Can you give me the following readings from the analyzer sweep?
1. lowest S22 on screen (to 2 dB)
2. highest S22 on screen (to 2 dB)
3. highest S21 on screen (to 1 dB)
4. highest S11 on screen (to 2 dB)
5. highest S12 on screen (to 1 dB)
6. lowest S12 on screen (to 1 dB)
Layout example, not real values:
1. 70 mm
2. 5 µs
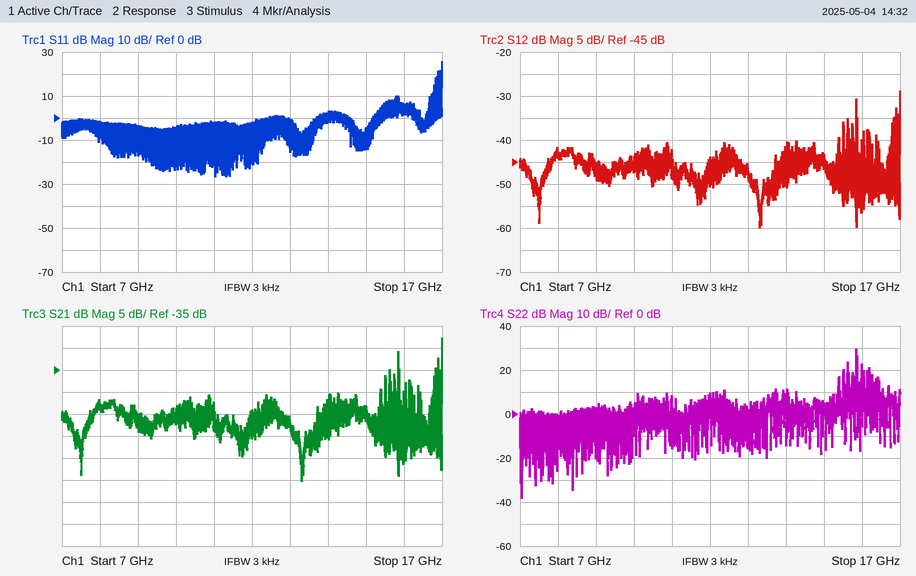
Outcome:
1. -38 dB
2. 30 dB
3. -28 dB
4. 26 dB
5. -29 dB
6. -60 dB
